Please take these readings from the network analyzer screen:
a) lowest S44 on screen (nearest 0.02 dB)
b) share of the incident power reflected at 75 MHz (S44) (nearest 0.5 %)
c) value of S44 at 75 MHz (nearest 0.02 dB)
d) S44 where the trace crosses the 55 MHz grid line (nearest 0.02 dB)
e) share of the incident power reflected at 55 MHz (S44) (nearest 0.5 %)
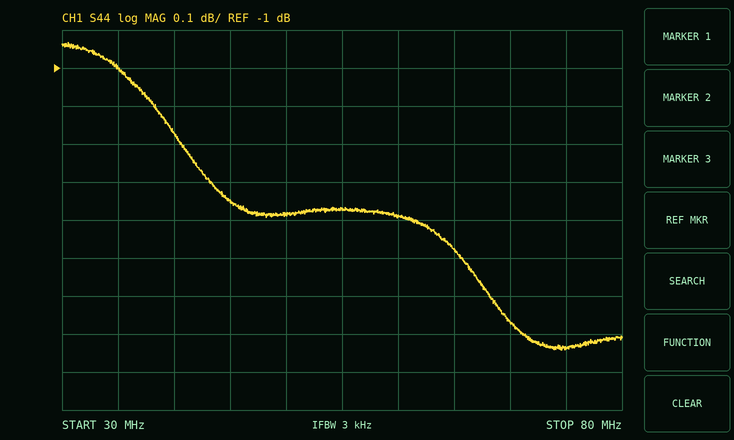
-1.74 dB
67.0 %
-1.74 dB
-1.38 dB
73.0 %
